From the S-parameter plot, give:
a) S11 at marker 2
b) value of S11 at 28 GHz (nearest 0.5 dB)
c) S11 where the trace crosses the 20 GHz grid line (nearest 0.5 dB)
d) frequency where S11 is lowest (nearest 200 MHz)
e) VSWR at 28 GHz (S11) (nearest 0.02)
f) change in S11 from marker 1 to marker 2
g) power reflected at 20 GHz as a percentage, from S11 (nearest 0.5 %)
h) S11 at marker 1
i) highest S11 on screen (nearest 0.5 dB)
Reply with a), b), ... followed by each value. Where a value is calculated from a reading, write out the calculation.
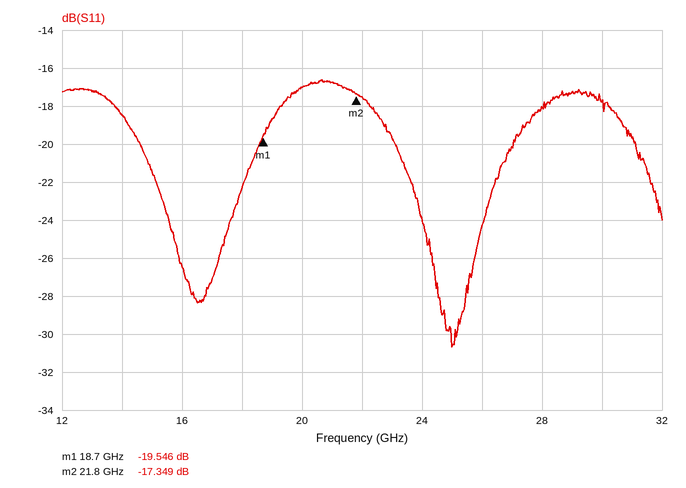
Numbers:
a) -17.349 dB
b) -18.0 dB
c) -17.0 dB
d) 25.0 GHz
e) |Γ| = 10^(-18/20) = 0.1259; VSWR = (1 + 0.1259)/(1 − 0.1259) ≈ 1.29, so 1.28 to the nearest 0.02
f) -17.349 − (-19.546) = 2.197 dB
g) 10^(-17/10) ≈ 2.0 %
h) -19.546 dB
i) -16.5 dB
